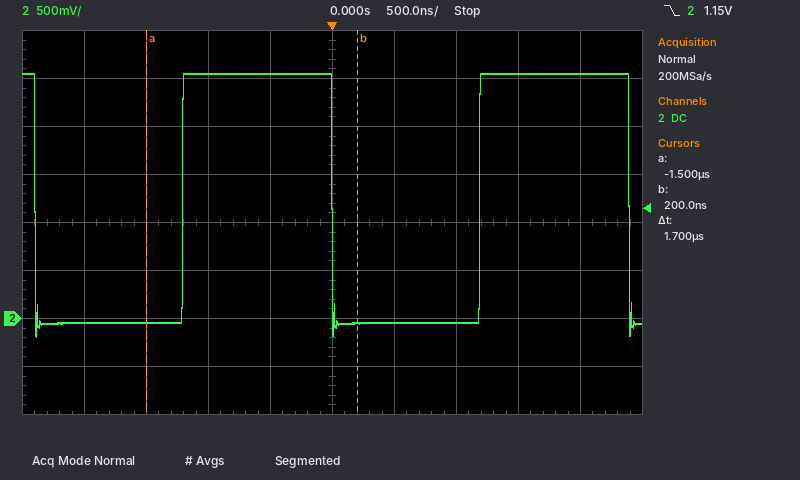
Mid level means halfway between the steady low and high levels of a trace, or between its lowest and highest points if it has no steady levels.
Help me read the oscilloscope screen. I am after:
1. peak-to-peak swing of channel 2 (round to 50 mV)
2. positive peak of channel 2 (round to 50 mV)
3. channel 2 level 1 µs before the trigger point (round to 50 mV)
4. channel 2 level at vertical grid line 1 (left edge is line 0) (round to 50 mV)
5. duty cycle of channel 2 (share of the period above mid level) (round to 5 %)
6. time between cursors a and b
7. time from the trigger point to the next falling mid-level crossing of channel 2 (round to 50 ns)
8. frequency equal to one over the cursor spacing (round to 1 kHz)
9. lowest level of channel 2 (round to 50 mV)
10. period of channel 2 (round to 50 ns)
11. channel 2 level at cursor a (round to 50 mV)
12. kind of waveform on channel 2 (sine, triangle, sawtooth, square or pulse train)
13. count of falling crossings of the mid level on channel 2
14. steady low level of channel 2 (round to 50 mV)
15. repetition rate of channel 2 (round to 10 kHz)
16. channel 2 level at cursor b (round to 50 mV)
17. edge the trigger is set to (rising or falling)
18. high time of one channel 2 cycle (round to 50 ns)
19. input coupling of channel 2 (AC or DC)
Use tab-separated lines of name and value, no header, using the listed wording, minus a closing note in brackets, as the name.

peak-to-peak swing of channel 2	2.75 V
positive peak of channel 2	2.55 V
channel 2 level 1 µs before the trigger point	2.55 V
channel 2 level at vertical grid line 1 (left edge is line 0)	-50 mV
duty cycle of channel 2 (share of the period above mid level)	50 %
time between cursors a and b	1.7 µs
time from the trigger point to the next falling mid-level crossing of channel 2	2.40 µs
frequency equal to one over the cursor spacing	588 kHz
lowest level of channel 2	-200 mV
period of channel 2	2.40 µs
channel 2 level at cursor a	-50 mV
kind of waveform on channel 2	square
count of falling crossings of the mid level on channel 2	3
steady low level of channel 2	-50 mV
repetition rate of channel 2	420 kHz
channel 2 level at cursor b	-50 mV
edge the trigger is set to	falling
high time of one channel 2 cycle	1.20 µs
input coupling of channel 2	DC
